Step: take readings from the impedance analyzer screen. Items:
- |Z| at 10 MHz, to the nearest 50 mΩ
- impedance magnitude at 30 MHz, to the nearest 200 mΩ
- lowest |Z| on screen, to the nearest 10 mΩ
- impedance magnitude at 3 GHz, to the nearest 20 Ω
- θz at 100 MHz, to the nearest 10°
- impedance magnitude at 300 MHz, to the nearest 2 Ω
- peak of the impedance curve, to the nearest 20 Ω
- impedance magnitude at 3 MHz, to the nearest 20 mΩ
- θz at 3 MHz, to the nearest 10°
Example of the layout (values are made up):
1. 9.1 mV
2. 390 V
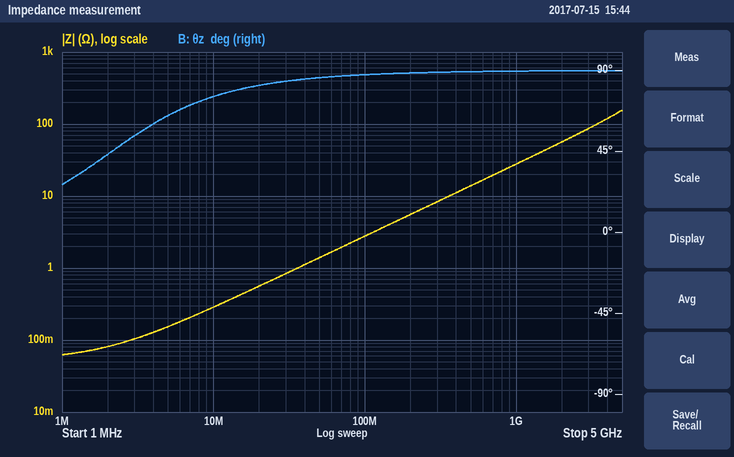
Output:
1. 300 mΩ
2. 800 mΩ
3. 60 mΩ
4. 80 Ω
5. 90°
6. 8 Ω
7. 160 Ω
8. 100 mΩ
9. 50°
